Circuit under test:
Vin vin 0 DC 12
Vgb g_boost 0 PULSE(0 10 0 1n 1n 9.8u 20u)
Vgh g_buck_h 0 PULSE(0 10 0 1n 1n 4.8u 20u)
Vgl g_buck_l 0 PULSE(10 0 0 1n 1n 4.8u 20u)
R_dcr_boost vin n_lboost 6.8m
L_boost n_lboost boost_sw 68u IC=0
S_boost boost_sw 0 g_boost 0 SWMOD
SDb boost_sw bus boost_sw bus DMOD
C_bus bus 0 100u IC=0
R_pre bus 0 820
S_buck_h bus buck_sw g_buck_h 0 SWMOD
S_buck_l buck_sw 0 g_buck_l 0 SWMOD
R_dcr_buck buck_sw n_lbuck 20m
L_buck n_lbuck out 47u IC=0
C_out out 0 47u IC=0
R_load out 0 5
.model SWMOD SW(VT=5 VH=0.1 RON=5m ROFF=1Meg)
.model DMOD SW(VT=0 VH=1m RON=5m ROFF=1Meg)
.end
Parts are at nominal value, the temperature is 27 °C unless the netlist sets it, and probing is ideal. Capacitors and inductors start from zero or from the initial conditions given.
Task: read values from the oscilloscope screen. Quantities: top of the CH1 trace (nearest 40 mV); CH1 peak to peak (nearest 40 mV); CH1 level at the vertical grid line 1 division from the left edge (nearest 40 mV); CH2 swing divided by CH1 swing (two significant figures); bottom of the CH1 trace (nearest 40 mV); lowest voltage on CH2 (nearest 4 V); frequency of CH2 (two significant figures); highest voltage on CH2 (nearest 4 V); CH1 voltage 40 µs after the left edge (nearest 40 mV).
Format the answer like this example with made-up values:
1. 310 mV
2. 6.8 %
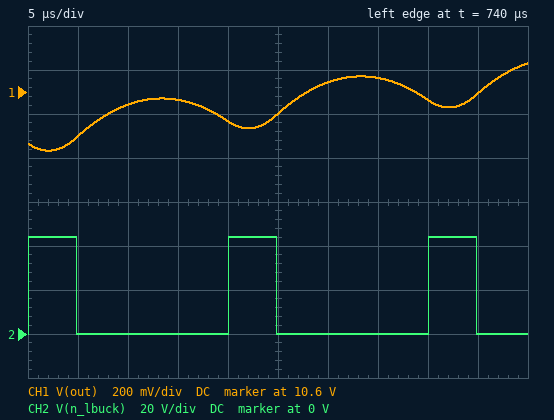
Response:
1. 10.72 V
2. 400 mV
3. 10.40 V
4. 110
5. 10.32 V
6. 0 V
7. 50 kHz
8. 44 V
9. 10.56 V
